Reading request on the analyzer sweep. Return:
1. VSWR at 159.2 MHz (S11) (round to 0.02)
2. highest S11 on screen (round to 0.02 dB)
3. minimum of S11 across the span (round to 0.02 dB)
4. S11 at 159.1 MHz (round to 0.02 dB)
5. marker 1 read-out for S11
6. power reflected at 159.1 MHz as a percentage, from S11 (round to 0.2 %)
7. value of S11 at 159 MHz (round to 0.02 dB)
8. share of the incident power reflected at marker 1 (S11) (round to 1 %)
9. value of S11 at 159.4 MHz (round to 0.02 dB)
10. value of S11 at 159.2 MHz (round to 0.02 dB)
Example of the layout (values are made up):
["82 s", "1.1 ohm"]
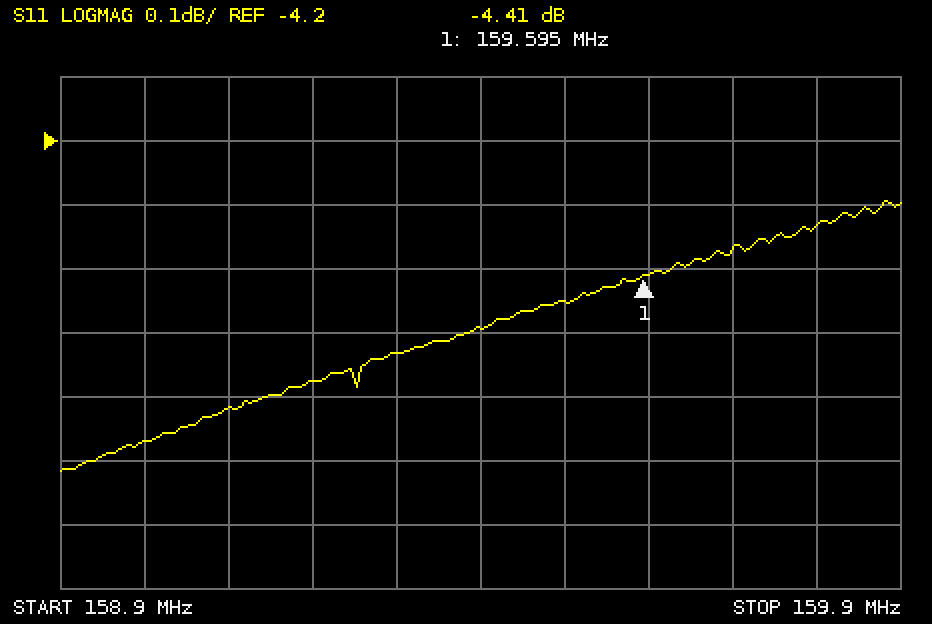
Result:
["3.88", "-4.30 dB", "-4.72 dB", "-4.62 dB", "-4.41 dB", "34.6 %", "-4.66 dB", "36 %", "-4.50 dB", "-4.58 dB"]
